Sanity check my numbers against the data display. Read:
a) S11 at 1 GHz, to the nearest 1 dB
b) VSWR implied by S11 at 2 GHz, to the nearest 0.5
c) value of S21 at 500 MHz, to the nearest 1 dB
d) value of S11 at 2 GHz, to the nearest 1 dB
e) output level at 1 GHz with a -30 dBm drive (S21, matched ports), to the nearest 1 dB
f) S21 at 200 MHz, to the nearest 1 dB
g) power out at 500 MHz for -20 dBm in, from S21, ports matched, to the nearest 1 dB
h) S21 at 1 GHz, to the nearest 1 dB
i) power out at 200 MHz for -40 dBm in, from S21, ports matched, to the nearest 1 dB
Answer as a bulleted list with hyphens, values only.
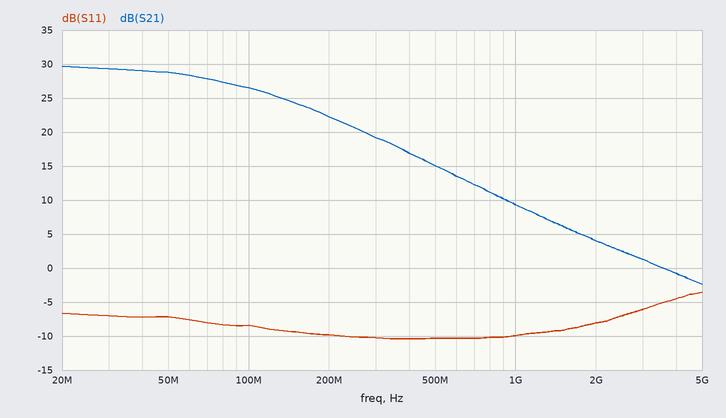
- -10 dB
- 2.5
- 15 dB
- -8 dB
- -21 dBm
- 22 dB
- -5 dBm
- 9 dB
- -18 dBm
